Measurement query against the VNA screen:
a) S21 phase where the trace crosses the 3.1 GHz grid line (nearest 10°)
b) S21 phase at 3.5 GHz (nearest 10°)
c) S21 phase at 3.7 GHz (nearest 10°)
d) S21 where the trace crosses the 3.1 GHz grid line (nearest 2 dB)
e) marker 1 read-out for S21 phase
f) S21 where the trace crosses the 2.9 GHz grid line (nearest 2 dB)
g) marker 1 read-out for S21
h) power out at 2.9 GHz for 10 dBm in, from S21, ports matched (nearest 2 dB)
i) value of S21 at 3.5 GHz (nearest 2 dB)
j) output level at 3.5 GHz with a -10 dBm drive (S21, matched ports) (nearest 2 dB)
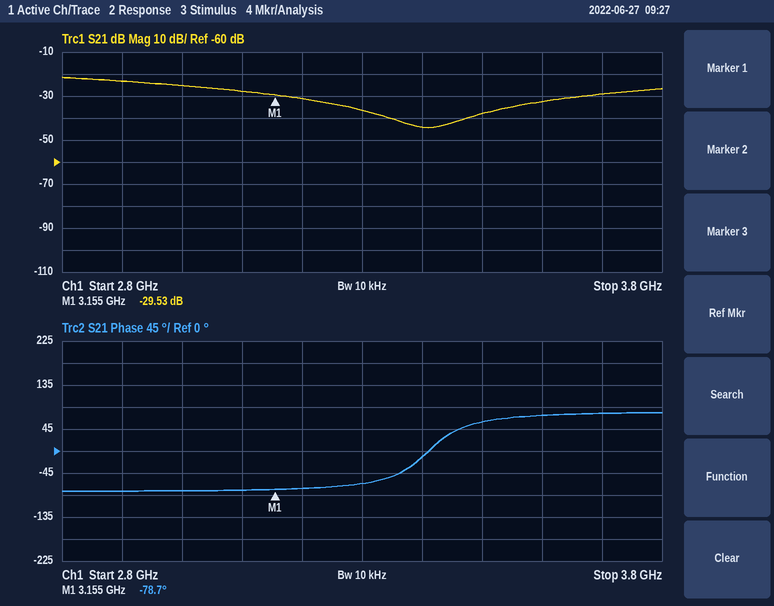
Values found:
-80°
60°
80°
-28 dB
-78.7°
-24 dB
-29.53 dB
-14 dBm
-38 dB
-48 dBm
